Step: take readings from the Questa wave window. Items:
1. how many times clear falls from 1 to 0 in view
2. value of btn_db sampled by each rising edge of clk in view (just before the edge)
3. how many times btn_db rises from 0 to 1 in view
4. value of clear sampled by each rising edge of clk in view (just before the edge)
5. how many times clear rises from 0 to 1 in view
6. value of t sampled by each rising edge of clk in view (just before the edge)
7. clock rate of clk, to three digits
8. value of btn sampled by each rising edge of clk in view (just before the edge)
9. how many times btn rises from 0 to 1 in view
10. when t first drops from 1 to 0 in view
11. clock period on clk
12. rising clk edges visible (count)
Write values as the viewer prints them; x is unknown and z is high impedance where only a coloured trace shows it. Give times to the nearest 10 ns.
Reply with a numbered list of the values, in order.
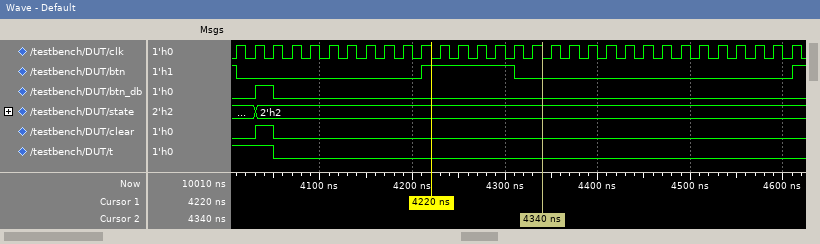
1. 1
2. 0 0 1 0 0 0 0 0 0 0 0 0 0 0 0 0 0 0 0 0 0 0 0 0 0 0 0 0 0 0 0
3. 1
4. 0 0 1 0 0 0 0 0 0 0 0 0 0 0 0 0 0 0 0 0 0 0 0 0 0 0 0 0 0 0 0
5. 1
6. 1 1 1 0 0 0 0 0 0 0 0 0 0 0 0 0 0 0 0 0 0 0 0 0 0 0 0 0 0 0 0
7. 50.0 MHz
8. 1 0 0 0 0 0 0 0 0 0 0 1 1 1 1 1 0 0 0 0 0 0 0 0 0 0 0 0 0 0 0
9. 2
10. 4050 ns
11. 20 ns
12. 31
